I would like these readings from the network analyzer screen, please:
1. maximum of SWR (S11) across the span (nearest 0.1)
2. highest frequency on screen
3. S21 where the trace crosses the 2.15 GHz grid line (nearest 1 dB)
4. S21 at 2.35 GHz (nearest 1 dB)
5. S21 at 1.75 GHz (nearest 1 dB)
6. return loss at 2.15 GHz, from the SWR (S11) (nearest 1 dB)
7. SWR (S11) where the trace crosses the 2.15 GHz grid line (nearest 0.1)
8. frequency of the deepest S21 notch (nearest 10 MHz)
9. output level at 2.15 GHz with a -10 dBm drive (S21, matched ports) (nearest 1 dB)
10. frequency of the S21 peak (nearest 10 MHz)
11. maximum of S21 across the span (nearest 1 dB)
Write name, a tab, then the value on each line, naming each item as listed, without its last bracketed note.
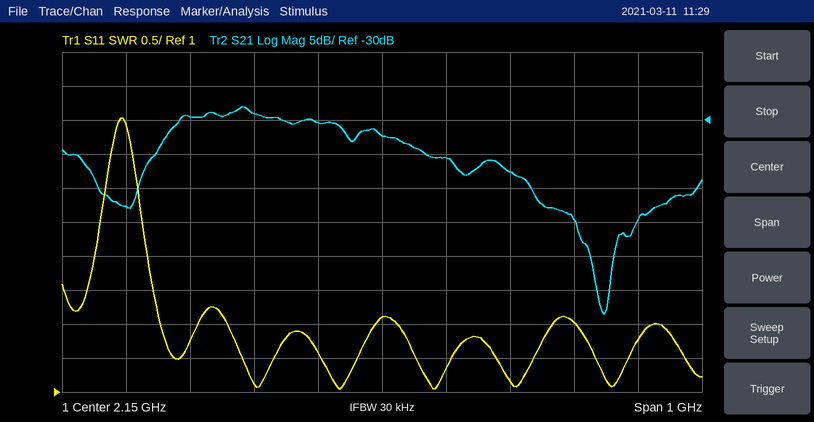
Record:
maximum of SWR (S11) across the span	5.0
highest frequency on screen	2.65 GHz
S21 where the trace crosses the 2.15 GHz grid line	-32 dB
S21 at 2.35 GHz	-38 dB
S21 at 1.75 GHz	-43 dB
return loss at 2.15 GHz, from the SWR (S11)	9 dB
SWR (S11) where the trace crosses the 2.15 GHz grid line	2.1
frequency of the deepest S21 notch	2.50 GHz
output level at 2.15 GHz with a -10 dBm drive (S21, matched ports)	-42 dBm
frequency of the S21 peak	1.93 GHz
maximum of S21 across the span	-28 dB
